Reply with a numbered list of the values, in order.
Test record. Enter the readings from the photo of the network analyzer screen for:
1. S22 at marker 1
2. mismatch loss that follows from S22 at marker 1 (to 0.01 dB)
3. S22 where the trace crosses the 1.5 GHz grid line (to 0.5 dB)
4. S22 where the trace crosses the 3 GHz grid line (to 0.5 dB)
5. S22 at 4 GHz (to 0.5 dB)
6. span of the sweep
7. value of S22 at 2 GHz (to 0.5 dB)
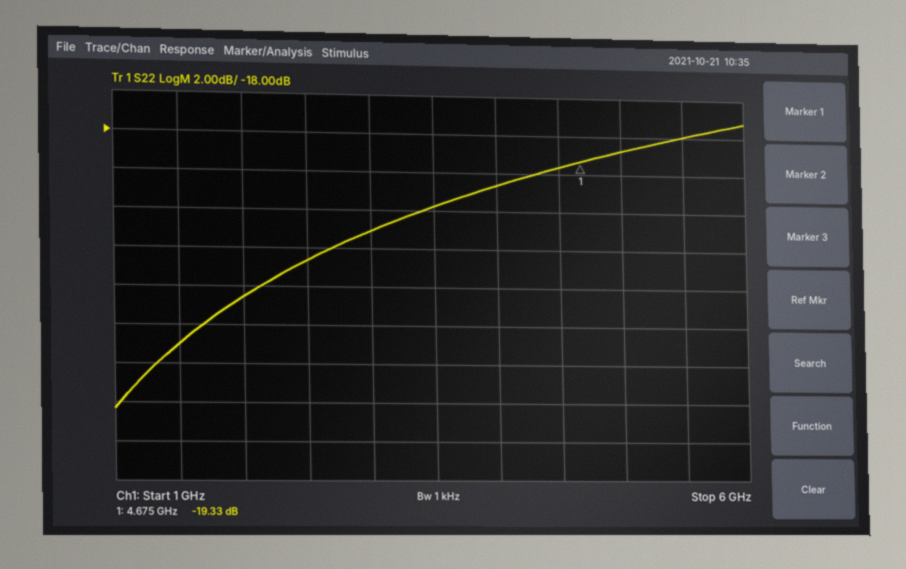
1. -19.33 dB
2. 0.05 dB
3. -29.0 dB
4. -23.0 dB
5. -20.5 dB
6. 5 GHz
7. -26.5 dB
